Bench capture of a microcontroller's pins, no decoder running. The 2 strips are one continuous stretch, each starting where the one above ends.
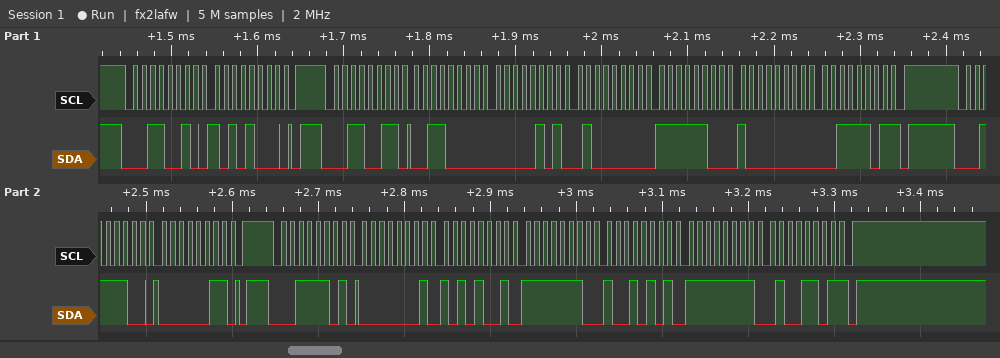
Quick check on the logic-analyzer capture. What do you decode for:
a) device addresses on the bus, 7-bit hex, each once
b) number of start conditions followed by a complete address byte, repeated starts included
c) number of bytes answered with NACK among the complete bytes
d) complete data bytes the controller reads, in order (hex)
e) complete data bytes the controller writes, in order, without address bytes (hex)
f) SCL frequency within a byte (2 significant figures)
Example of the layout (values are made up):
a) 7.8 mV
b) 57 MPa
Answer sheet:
a) 0x19 0x1E
b) 4
c) 2
d) 30 05 40 FC 80 3D 01 A9 FE 95 FF 4D
e) A8 03
f) 100 kHz
